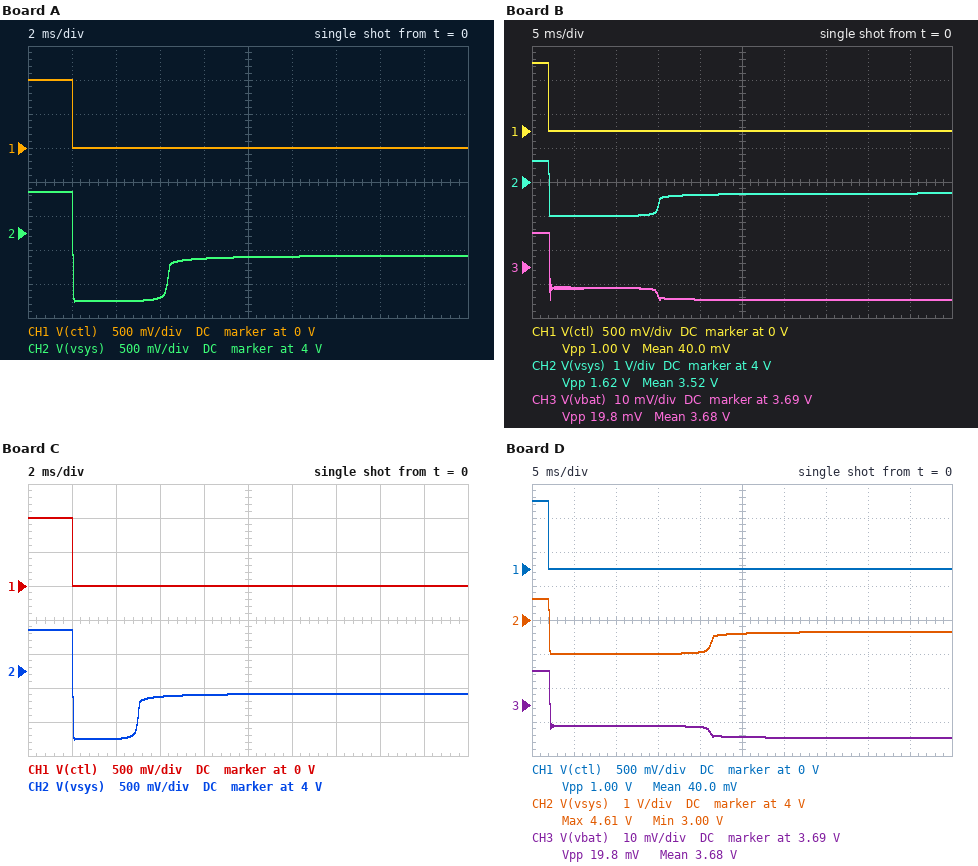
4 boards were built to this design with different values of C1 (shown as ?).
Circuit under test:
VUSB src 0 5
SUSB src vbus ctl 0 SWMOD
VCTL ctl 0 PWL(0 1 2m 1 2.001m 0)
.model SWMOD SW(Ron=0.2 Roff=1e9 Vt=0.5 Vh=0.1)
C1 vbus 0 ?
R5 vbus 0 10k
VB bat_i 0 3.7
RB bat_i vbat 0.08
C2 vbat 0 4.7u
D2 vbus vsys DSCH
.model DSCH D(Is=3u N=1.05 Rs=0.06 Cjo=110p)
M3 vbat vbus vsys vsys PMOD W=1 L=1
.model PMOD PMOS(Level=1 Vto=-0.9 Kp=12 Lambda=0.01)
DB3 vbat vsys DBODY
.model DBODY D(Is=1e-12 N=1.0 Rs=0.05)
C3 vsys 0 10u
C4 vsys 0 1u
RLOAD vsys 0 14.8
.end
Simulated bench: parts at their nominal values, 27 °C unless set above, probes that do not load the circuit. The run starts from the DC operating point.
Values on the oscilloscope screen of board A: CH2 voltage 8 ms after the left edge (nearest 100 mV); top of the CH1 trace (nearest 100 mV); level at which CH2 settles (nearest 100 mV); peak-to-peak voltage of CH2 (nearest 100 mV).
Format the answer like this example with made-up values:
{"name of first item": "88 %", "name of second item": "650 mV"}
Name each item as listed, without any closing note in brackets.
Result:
{"CH2 voltage 8 ms after the left edge": "3.6 V", "top of the CH1 trace": "1.0 V", "level at which CH2 settles": "3.7 V", "peak-to-peak voltage of CH2": "1.6 V"}
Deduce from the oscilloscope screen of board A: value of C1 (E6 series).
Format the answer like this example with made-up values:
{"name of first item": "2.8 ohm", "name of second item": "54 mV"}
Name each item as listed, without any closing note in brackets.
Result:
{"value of C1": "2.2 µF"}
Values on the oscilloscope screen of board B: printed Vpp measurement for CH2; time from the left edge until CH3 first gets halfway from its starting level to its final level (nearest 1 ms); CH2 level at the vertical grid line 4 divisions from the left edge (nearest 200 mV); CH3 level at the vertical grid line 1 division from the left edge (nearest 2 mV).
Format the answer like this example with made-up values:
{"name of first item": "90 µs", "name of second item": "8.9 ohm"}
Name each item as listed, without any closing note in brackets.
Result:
{"printed Vpp measurement for CH2": "1.62 V", "time from the left edge until CH3 first gets halfway from its starting level to its final level": "2 ms", "CH2 level at the vertical grid line 4 divisions from the left edge": "3.6 V", "CH3 level at the vertical grid line 1 division from the left edge": "3.684 V"}
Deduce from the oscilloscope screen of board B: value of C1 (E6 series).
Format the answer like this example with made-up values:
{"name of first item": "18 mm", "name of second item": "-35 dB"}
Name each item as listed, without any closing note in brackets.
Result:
{"value of C1": "6.8 µF"}
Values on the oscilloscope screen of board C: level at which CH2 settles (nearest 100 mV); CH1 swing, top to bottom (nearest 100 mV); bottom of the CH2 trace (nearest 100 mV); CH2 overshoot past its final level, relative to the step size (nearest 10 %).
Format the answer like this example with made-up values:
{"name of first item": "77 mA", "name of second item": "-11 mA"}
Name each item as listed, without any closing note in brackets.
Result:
{"level at which CH2 settles": "3.7 V", "CH1 swing, top to bottom": "1.0 V", "bottom of the CH2 trace": "3.0 V", "CH2 overshoot past its final level, relative to the step size": "70 %"}
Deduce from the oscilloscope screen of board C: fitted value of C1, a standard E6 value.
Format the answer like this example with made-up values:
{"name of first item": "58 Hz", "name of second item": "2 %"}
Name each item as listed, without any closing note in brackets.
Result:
{"fitted value of C1, a standard E6 value": "1.5 µF"}
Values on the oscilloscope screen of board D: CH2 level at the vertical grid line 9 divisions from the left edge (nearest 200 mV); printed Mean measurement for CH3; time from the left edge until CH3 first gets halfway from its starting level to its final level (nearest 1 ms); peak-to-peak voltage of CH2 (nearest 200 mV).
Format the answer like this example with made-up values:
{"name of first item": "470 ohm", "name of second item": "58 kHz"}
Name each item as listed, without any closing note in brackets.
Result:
{"CH2 level at the vertical grid line 9 divisions from the left edge": "3.6 V", "printed Mean measurement for CH3": "3.68 V", "time from the left edge until CH3 first gets halfway from its starting level to its final level": "2 ms", "peak-to-peak voltage of CH2": "1.6 V"}
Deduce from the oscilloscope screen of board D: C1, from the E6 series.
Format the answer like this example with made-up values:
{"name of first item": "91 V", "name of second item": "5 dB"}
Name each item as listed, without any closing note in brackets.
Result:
{"C1, from the E6 series": "10 µF"}
